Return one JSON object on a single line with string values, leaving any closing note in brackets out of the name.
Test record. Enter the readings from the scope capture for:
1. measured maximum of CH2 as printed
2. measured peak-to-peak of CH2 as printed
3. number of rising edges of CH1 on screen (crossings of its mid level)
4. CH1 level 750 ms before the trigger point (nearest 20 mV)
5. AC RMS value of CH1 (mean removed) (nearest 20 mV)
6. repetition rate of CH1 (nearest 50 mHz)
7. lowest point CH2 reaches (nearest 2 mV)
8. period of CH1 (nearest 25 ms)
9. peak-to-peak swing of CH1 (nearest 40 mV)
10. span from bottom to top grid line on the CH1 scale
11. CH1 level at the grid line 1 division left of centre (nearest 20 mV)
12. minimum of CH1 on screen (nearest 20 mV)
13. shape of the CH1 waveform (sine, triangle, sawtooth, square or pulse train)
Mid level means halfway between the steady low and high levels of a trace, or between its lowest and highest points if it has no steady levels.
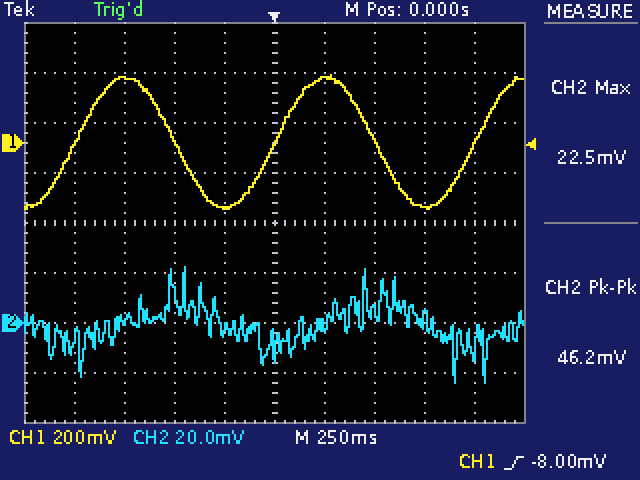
{"measured maximum of CH2 as printed": "22.5 mV", "measured peak-to-peak of CH2 as printed": "46.2 mV", "number of rising edges of CH1 on screen": "3", "CH1 level 750 ms before the trigger point": "260 mV", "AC RMS value of CH1 (mean removed)": "180 mV", "repetition rate of CH1": "1.00 Hz", "lowest point CH2 reaches": "-24 mV", "period of CH1": "1.000 s", "peak-to-peak swing of CH1": "520 mV", "span from bottom to top grid line on the CH1 scale": "1.6 V", "CH1 level at the grid line 1 division left of centre": "-260 mV", "minimum of CH1 on screen": "-260 mV", "shape of the CH1 waveform": "sine"}
